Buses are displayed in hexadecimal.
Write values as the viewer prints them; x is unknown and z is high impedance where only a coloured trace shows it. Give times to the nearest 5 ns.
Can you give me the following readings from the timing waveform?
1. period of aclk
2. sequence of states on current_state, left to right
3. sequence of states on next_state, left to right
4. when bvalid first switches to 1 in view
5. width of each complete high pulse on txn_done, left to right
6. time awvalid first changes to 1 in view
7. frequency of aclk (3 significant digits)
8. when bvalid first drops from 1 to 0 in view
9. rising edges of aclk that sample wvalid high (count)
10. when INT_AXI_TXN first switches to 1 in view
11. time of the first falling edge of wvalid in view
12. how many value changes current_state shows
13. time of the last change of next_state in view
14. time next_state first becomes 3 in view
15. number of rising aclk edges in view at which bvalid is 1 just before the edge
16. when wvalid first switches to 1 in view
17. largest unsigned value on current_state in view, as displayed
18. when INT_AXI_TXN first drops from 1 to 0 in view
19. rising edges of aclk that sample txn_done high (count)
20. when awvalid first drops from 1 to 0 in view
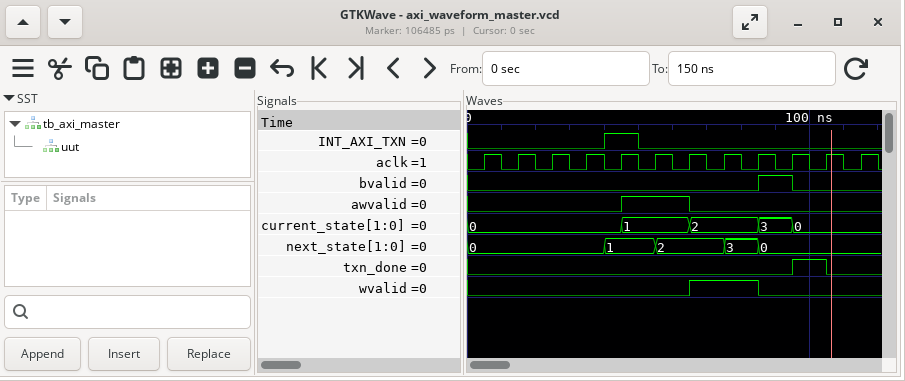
10 ns
0, 1, 2, 3, 0
0, 1, 2, 3, 0
85 ns
10 ns
45 ns
100 MHz
95 ns
2
40 ns
85 ns
4
85 ns
75 ns
1
65 ns
3
50 ns
1
65 ns
